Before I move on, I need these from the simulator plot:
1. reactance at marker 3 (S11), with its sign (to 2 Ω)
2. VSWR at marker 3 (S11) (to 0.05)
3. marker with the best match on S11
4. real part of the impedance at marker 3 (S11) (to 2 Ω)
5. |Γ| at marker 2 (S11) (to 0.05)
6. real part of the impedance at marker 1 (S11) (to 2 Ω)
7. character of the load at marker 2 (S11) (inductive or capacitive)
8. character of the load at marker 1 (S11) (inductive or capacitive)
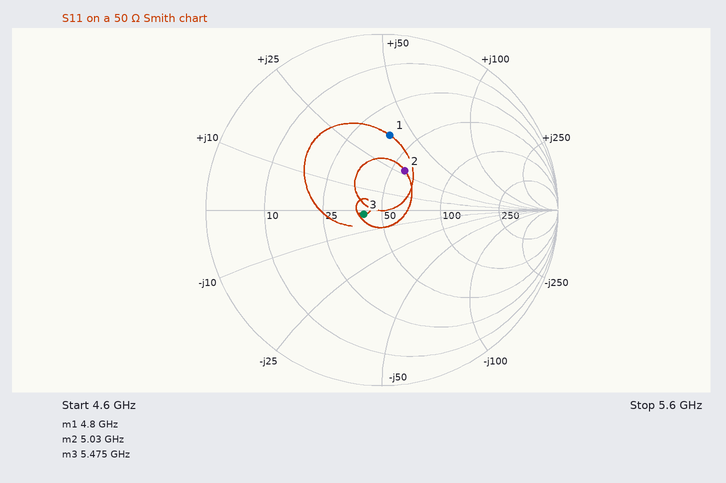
-2 Ω
1.25
marker 3
40 Ω
0.25
38 Ω
inductive
inductive
